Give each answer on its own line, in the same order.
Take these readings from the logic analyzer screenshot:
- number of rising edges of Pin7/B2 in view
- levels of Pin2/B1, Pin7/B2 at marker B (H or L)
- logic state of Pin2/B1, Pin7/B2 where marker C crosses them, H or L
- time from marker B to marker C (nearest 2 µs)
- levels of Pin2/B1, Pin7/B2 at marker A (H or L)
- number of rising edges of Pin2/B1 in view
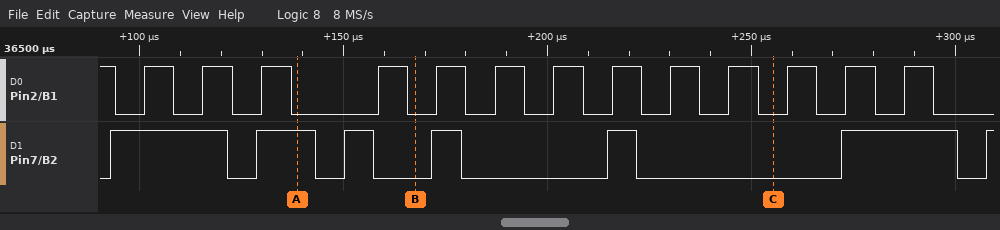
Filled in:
7
Pin2/B1=L, Pin7/B2=L
Pin2/B1=L, Pin7/B2=L
88 µs
Pin2/B1=L, Pin7/B2=H
13
